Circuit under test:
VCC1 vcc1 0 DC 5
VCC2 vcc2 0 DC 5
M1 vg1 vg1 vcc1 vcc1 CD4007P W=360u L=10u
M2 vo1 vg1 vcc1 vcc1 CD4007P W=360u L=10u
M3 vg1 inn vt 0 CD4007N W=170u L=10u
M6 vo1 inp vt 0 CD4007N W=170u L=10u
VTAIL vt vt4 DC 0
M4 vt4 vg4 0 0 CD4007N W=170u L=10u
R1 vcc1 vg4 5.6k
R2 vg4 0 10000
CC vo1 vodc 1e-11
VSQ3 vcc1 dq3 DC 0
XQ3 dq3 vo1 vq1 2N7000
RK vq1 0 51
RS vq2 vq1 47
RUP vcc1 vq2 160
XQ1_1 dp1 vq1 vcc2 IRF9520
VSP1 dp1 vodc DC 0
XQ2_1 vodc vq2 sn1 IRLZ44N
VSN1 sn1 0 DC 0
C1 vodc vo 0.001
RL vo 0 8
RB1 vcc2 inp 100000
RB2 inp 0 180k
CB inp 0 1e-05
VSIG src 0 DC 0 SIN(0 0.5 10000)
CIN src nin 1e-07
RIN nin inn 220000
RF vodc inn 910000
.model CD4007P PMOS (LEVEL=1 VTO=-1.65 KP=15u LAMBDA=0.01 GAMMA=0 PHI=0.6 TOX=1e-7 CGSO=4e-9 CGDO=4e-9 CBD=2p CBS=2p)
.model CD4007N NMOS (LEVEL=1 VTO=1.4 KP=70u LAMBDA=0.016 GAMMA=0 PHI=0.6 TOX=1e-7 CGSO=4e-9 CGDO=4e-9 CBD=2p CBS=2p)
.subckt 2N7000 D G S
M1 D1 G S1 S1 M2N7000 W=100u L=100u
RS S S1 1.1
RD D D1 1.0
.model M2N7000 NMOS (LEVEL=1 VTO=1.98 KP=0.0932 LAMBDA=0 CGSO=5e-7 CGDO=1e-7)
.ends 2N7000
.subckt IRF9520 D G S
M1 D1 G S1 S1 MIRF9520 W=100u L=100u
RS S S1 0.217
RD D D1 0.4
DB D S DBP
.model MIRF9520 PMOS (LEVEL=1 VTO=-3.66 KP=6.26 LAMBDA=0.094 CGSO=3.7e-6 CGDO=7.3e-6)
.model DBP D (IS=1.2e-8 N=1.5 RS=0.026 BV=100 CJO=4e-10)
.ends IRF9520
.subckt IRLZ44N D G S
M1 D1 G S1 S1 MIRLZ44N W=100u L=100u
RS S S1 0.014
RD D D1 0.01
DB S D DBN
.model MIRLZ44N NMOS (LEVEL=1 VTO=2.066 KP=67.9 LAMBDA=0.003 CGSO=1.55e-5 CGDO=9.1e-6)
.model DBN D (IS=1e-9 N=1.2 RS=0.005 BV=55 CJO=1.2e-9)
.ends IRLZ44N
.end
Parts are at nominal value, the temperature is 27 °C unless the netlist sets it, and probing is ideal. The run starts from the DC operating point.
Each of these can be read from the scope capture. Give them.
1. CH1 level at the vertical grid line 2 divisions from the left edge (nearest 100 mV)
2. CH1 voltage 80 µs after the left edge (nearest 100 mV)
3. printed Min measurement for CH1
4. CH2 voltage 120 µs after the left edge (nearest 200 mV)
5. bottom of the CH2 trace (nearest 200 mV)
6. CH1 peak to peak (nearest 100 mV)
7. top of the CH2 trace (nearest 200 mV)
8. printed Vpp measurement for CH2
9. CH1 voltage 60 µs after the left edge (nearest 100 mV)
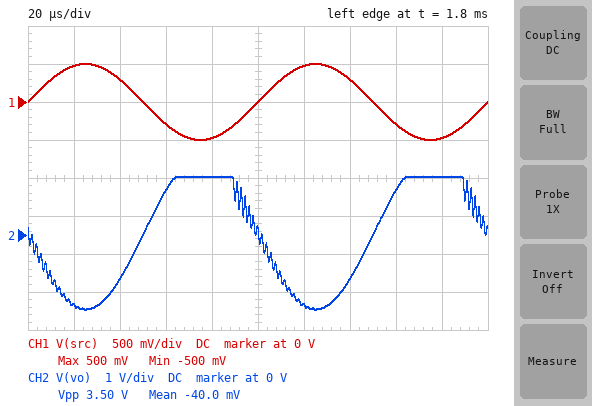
300 mV
-500 mV
-500 mV
-1.8 V
-2.0 V
1.0 V
1.6 V
3.50 V
-300 mV
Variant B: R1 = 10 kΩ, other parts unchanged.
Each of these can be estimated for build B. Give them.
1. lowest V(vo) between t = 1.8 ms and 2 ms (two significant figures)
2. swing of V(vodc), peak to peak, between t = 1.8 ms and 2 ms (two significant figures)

-3.2 V
4.7 V
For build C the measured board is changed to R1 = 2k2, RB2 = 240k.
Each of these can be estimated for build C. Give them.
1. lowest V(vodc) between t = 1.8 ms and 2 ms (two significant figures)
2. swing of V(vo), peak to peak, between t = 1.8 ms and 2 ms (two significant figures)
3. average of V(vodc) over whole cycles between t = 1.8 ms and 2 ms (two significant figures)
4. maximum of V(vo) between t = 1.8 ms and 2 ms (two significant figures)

3.8 V
1.2 V
4.5 V
290 mV
